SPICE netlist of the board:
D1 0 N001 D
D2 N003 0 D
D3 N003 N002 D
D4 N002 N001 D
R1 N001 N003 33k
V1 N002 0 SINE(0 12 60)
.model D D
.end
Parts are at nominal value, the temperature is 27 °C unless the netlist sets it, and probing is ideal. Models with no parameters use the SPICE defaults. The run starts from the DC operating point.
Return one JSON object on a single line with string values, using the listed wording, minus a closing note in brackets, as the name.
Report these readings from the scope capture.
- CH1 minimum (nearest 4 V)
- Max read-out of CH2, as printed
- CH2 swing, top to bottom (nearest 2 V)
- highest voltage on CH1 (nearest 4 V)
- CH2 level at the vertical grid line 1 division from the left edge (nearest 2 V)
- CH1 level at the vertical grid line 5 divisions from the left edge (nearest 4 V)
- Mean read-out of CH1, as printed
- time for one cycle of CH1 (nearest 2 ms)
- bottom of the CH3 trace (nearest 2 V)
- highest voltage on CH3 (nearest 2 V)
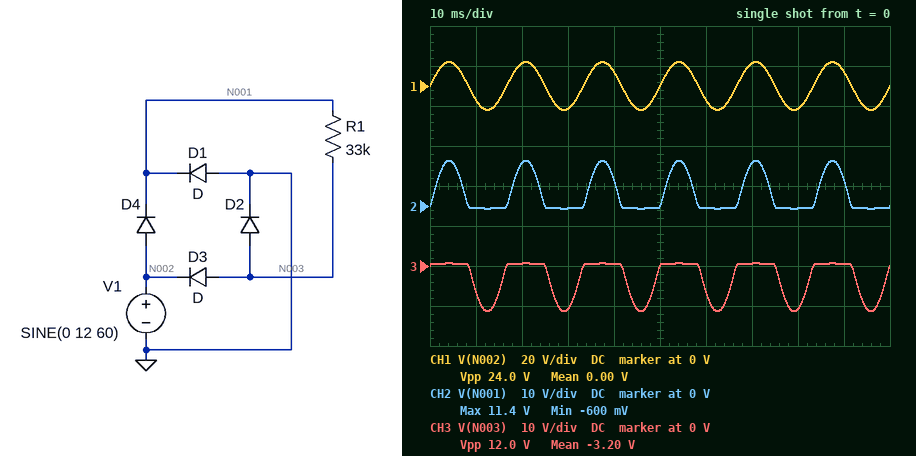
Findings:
{"CH1 minimum": "-12 V", "Max read-out of CH2, as printed": "11.4 V", "CH2 swing, top to bottom": "12 V", "highest voltage on CH1": "12 V", "CH2 level at the vertical grid line 1 division from the left edge": "0 V", "CH1 level at the vertical grid line 5 divisions from the left edge": "0 V", "Mean read-out of CH1, as printed": "0.00 V", "time for one cycle of CH1": "16 ms", "bottom of the CH3 trace": "-12 V", "highest voltage on CH3": "0 V"}
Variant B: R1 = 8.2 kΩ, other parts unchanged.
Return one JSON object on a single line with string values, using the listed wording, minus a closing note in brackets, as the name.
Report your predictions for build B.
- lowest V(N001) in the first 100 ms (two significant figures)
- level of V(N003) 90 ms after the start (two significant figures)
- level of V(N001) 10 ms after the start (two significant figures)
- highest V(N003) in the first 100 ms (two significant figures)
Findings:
{"lowest V(N001) in the first 100 ms": "-660 mV", "level of V(N003) 90 ms after the start": "650 mV", "level of V(N001) 10 ms after the start": "-650 mV", "highest V(N003) in the first 100 ms": "660 mV"}
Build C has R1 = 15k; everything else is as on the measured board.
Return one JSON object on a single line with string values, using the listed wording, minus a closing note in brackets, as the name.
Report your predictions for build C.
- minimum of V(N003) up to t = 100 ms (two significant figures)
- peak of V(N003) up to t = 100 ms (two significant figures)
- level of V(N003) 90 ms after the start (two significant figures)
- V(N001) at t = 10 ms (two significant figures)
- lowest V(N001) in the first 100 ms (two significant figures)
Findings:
{"minimum of V(N003) up to t = 100 ms": "-11 V", "peak of V(N003) up to t = 100 ms": "650 mV", "level of V(N003) 90 ms after the start": "630 mV", "V(N001) at t = 10 ms": "-630 mV", "lowest V(N001) in the first 100 ms": "-650 mV"}
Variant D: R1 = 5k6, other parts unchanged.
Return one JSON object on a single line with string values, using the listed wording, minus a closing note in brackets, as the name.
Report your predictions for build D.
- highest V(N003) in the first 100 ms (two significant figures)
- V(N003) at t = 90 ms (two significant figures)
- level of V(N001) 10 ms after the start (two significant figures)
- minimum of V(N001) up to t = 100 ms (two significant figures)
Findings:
{"highest V(N003) in the first 100 ms": "670 mV", "V(N003) at t = 90 ms": "660 mV", "level of V(N001) 10 ms after the start": "-660 mV", "minimum of V(N001) up to t = 100 ms": "-670 mV"}
